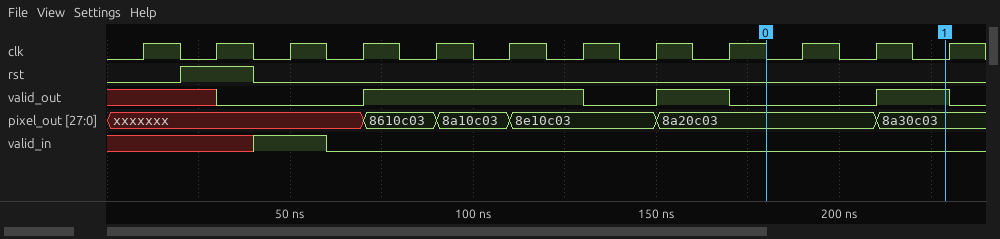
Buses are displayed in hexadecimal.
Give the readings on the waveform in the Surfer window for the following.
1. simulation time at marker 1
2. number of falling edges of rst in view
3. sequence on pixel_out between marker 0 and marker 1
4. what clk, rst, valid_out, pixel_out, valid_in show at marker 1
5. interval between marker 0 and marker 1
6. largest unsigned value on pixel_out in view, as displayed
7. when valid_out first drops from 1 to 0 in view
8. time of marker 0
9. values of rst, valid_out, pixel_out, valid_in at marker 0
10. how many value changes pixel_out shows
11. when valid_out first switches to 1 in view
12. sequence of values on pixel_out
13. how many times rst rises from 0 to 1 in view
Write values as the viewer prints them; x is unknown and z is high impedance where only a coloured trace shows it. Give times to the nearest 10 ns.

230 ns
1
8a20c03, 8a30c03
clk=0, rst=0, valid_out=1, pixel_out=8a30c03, valid_in=0
50 ns
8e10c03
130 ns
180 ns
rst=0, valid_out=0, pixel_out=8a20c03, valid_in=0
5
70 ns
xxxxxxx, 8610c03, 8a10c03, 8e10c03, 8a20c03, 8a30c03
1
